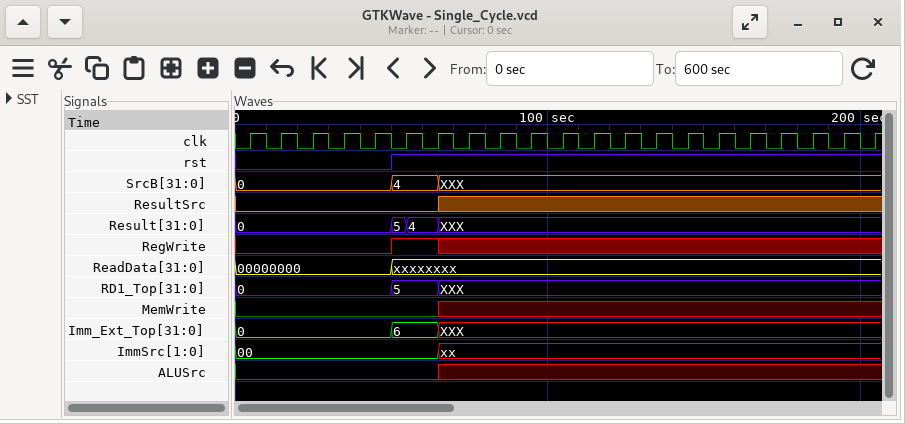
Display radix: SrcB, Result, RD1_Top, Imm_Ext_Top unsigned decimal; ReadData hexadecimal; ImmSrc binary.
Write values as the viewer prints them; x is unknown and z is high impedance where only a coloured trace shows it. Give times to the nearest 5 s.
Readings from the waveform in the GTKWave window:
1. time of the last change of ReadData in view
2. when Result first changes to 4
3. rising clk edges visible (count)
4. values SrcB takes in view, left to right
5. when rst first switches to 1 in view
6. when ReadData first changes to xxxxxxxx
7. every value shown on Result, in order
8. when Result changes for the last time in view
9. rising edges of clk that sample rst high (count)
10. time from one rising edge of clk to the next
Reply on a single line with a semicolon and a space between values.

50 s; 55 s; 21; 0, 4, XXX; 50 s; 50 s; 0, 5, 4, XXX; 65 s; 16; 10 s
